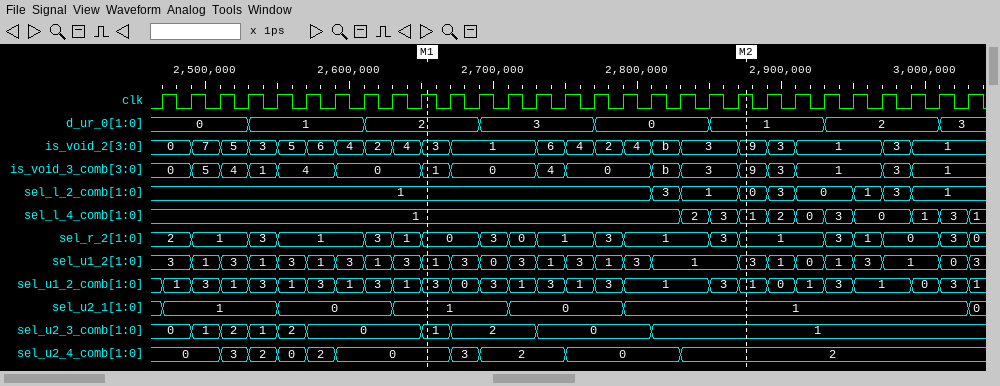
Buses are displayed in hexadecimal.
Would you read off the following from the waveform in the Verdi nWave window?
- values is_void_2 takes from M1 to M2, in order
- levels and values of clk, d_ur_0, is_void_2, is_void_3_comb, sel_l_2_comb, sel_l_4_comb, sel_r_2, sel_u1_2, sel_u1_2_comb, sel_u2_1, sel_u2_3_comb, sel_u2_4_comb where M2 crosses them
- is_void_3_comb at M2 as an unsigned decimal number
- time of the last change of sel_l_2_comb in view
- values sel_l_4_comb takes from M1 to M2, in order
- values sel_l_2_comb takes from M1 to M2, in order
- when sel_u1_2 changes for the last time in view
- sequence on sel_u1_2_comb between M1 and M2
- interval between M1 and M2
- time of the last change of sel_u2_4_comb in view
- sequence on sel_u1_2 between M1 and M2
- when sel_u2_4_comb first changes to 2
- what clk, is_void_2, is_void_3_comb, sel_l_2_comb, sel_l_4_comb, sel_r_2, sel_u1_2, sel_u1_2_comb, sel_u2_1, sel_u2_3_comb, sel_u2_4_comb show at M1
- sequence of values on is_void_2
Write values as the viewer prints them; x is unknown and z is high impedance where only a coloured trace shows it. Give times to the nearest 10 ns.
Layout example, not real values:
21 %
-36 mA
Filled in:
3, 1, 6, 4, 2, 4, b, 3, 9
clk=1, d_ur_0=1, is_void_2=9, is_void_3_comb=9, sel_l_2_comb=0, sel_l_4_comb=1, sel_r_2=1, sel_u1_2=3, sel_u1_2_comb=1, sel_u2_1=1, sel_u2_3_comb=1, sel_u2_4_comb=2
9
2990 ns
1, 2, 3, 1
1, 3, 1, 0
3030 ns
3, 0, 3, 1, 3, 1, 3, 1, 3, 1
220 ns
2830 ns
1, 3, 0, 3, 1, 3, 1, 3, 1, 3
2530 ns
clk=1, is_void_2=3, is_void_3_comb=1, sel_l_2_comb=1, sel_l_4_comb=1, sel_r_2=0, sel_u1_2=1, sel_u1_2_comb=3, sel_u2_1=1, sel_u2_3_comb=1, sel_u2_4_comb=0
0, 7, 5, 3, 5, 6, 4, 2, 4, 3, 1, 6, 4, 2, 4, b, 3, 9, 3, 1, 3, 1
